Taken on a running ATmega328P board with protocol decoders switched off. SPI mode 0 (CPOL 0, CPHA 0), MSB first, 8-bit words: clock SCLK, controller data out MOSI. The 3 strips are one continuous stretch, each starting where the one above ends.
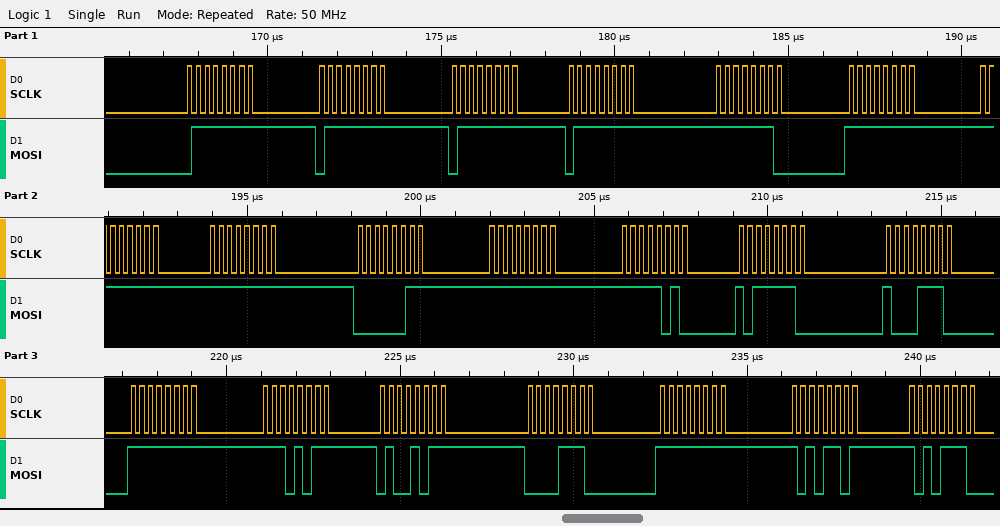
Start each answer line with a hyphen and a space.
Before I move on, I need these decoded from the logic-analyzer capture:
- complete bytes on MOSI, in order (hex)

- 7F 7F 7F 7F FE FF FF FF 03 FF FA BE 8E FF EB 4B 0E FF AD AE
